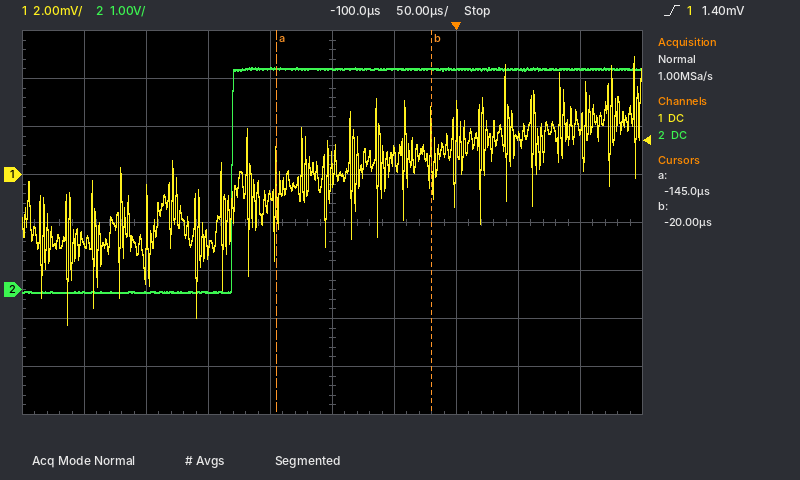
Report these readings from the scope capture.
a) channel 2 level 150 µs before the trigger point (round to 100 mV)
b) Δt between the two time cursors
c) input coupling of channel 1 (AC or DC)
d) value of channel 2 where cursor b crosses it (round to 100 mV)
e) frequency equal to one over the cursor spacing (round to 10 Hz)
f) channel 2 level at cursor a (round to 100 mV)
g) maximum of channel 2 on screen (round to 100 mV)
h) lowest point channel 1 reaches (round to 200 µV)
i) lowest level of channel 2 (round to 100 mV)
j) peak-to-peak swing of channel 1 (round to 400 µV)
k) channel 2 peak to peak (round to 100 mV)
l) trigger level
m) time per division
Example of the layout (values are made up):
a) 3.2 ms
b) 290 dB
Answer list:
a) 4.6 V
b) 125 µs
c) DC
d) 4.6 V
e) 8.00 kHz
f) 4.6 V
g) 4.6 V
h) -6.2 mV
i) -100 mV
j) 11.2 mV
k) 4.7 V
l) 1.40 mV
m) 50 µs
